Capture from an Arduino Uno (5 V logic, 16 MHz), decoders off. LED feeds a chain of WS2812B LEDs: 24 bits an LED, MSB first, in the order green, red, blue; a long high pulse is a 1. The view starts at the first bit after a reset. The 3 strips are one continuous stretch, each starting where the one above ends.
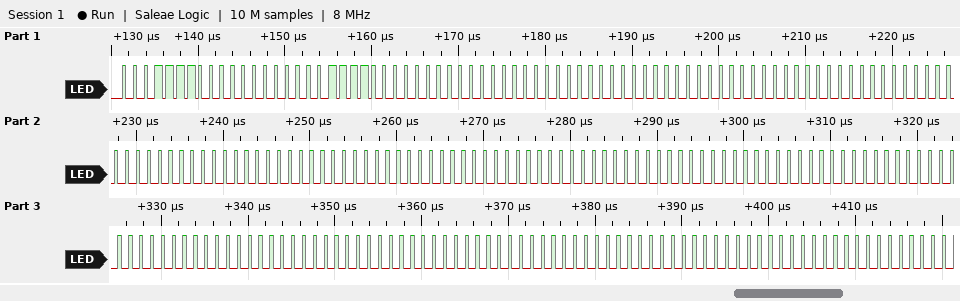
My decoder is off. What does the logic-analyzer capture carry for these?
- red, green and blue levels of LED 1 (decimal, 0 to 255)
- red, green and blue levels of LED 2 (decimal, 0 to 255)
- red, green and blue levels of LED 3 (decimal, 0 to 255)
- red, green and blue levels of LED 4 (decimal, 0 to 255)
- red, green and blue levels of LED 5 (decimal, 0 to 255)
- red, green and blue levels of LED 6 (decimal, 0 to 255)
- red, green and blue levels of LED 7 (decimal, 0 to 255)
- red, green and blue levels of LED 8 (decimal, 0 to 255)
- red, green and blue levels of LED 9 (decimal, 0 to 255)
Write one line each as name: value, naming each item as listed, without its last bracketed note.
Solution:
red, green and blue levels of LED 1: 0, 30, 30
red, green and blue levels of LED 2: 0, 0, 0
red, green and blue levels of LED 3: 0, 0, 0
red, green and blue levels of LED 4: 0, 0, 0
red, green and blue levels of LED 5: 0, 0, 0
red, green and blue levels of LED 6: 0, 0, 0
red, green and blue levels of LED 7: 0, 0, 0
red, green and blue levels of LED 8: 0, 0, 0
red, green and blue levels of LED 9: 0, 0, 0
